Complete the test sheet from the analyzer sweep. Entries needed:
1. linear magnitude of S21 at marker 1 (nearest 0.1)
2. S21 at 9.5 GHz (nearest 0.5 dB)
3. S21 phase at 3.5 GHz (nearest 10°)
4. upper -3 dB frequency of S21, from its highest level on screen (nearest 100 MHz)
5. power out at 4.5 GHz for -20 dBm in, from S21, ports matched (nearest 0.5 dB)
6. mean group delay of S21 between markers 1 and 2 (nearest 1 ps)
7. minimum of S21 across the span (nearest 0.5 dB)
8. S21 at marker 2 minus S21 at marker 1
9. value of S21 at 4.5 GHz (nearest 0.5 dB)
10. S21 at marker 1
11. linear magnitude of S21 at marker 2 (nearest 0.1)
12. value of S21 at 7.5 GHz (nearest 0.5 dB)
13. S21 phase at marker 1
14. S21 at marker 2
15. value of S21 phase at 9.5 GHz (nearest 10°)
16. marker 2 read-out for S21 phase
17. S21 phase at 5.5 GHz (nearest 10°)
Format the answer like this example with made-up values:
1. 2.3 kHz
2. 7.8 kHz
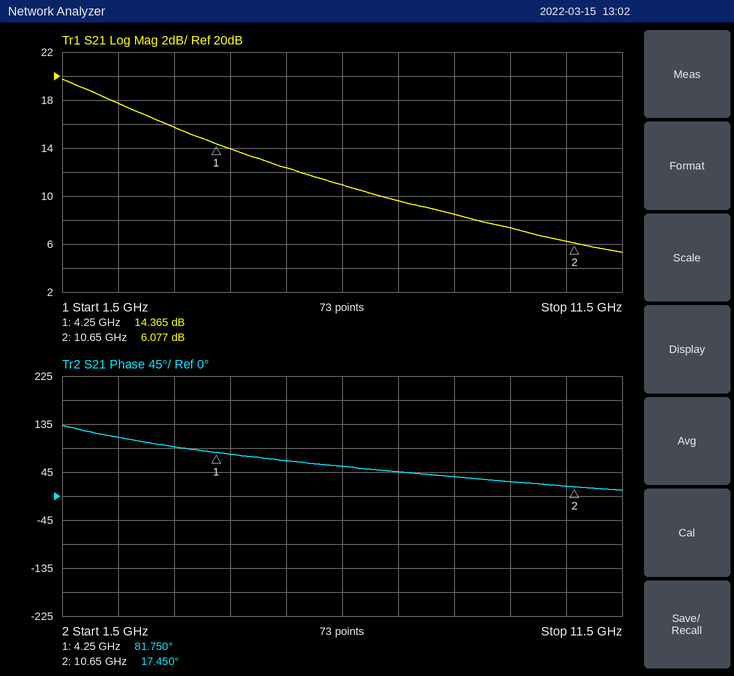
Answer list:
1. 5.2
2. 7.5 dB
3. 90°
4. 3.0 GHz
5. -6.0 dBm
6. 28 ps
7. 5.5 dB
8. -8.288 dB
9. 14.0 dB
10. 14.365 dB
11. 2.0
12. 9.5 dB
13. 81.750°
14. 6.077 dB
15. 30°
16. 17.450°
17. 70°
